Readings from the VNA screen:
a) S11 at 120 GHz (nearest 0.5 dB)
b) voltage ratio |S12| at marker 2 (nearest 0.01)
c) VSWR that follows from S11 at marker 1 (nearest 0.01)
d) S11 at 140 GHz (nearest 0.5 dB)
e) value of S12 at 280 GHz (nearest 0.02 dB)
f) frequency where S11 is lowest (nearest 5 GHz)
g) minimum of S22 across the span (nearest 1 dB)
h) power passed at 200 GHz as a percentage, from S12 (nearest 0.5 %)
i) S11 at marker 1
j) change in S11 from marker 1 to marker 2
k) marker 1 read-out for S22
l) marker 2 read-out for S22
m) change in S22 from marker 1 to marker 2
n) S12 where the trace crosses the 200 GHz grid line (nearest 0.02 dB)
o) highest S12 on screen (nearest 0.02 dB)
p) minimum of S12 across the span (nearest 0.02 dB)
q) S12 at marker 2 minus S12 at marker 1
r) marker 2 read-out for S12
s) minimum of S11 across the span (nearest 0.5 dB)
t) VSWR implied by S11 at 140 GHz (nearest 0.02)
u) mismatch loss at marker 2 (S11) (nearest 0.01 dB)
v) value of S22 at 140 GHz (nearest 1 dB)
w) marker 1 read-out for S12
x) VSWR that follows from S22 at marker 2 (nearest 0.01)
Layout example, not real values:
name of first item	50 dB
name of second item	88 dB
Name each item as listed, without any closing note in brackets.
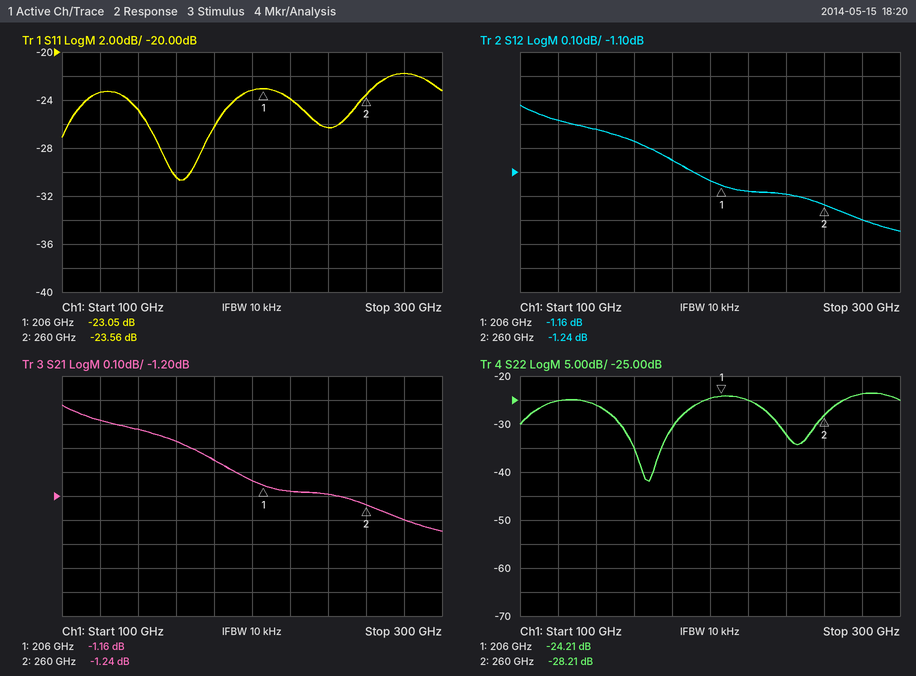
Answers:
S11 at 120 GHz	-23.5 dB
voltage ratio |S12| at marker 2	0.87
VSWR that follows from S11 at marker 1	1.15
S11 at 140 GHz	-25.0 dB
value of S12 at 280 GHz	-1.30 dB
frequency where S11 is lowest	160 GHz
minimum of S22 across the span	-42 dB
power passed at 200 GHz as a percentage, from S12	77.0 %
S11 at marker 1	-23.05 dB
change in S11 from marker 1 to marker 2	-0.51 dB
marker 1 read-out for S22	-24.21 dB
marker 2 read-out for S22	-28.21 dB
change in S22 from marker 1 to marker 2	-4.00 dB
S12 where the trace crosses the 200 GHz grid line	-1.14 dB
highest S12 on screen	-0.82 dB
minimum of S12 across the span	-1.34 dB
S12 at marker 2 minus S12 at marker 1	-0.08 dB
marker 2 read-out for S12	-1.24 dB
minimum of S11 across the span	-30.5 dB
VSWR implied by S11 at 140 GHz	1.12
mismatch loss at marker 2 (S11)	0.02 dB
value of S22 at 140 GHz	-26 dB
marker 1 read-out for S12	-1.16 dB
VSWR that follows from S22 at marker 2	1.08
